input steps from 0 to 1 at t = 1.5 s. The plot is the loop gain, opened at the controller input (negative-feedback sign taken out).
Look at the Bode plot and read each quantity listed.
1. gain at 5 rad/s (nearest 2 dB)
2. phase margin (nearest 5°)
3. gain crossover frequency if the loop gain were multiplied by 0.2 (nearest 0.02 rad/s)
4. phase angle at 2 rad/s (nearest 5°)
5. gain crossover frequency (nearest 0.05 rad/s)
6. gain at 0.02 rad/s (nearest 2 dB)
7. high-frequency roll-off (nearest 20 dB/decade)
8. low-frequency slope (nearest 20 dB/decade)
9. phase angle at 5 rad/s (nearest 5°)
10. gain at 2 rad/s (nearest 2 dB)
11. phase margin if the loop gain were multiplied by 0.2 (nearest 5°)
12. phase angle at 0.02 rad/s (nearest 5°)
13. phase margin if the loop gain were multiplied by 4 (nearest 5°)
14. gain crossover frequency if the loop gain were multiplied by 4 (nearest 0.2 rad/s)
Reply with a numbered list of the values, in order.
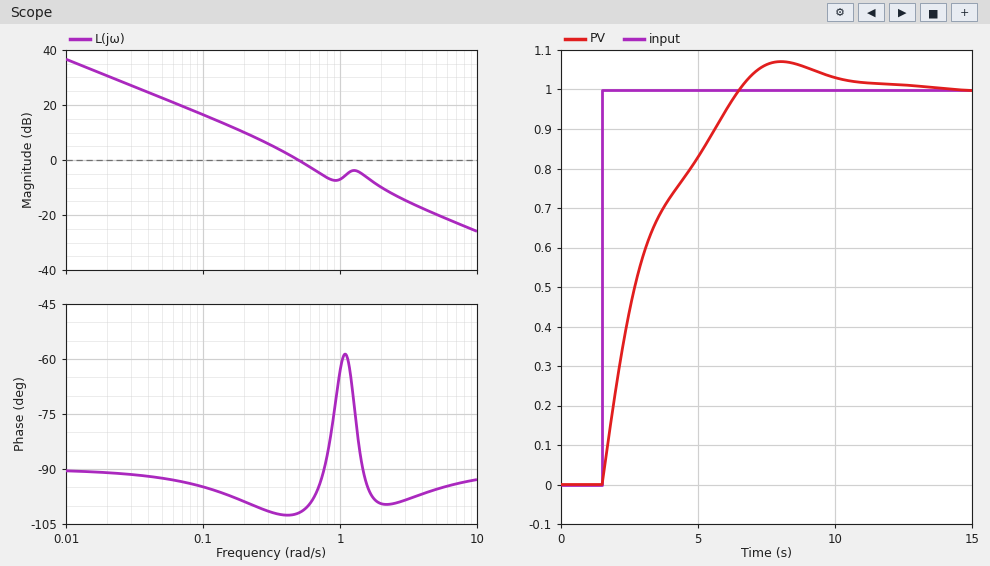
1. -20 dB
2. 80°
3. 0.14 rad/s
4. -100°
5. 0.50 rad/s
6. 30 dB
7. -20 dB/decade
8. -20 dB/decade
9. -95°
10. -10 dB
11. 85°
12. -90°
13. 80°
14. 2.4 rad/s
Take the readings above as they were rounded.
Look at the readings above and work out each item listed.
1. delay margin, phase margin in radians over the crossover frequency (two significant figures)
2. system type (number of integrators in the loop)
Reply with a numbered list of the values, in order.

1. 2.8 s
2. 1
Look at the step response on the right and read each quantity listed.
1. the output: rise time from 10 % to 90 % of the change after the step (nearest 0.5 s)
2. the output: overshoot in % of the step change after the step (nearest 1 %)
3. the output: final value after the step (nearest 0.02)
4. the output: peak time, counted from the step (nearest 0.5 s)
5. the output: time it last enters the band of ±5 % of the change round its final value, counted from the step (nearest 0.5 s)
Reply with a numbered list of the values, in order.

1. 4.0 s
2. 7 %
3. 1.00
4. 6.5 s
5. 7.5 s
